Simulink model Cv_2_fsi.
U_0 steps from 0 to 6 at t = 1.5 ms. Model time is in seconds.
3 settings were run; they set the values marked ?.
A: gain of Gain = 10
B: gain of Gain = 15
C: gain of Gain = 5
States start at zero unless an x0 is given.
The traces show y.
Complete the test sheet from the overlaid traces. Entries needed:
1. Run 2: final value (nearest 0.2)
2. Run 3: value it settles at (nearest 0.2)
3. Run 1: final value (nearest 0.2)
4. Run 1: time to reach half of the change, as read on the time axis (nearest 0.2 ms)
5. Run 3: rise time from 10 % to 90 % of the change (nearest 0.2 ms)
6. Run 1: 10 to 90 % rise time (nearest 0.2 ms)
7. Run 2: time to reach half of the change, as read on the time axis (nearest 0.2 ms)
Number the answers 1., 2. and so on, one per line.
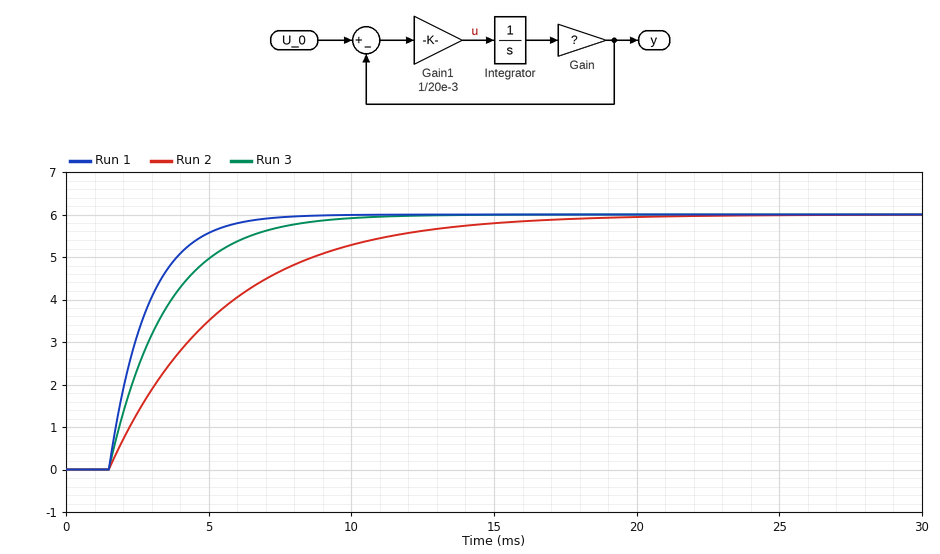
1. 6.0
2. 6.0
3. 6.0
4. 2.4 ms
5. 4.4 ms
6. 3.0 ms
7. 4.2 ms
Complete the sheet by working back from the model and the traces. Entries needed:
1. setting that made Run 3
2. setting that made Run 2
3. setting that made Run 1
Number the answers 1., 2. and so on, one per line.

1. A
2. C
3. B
